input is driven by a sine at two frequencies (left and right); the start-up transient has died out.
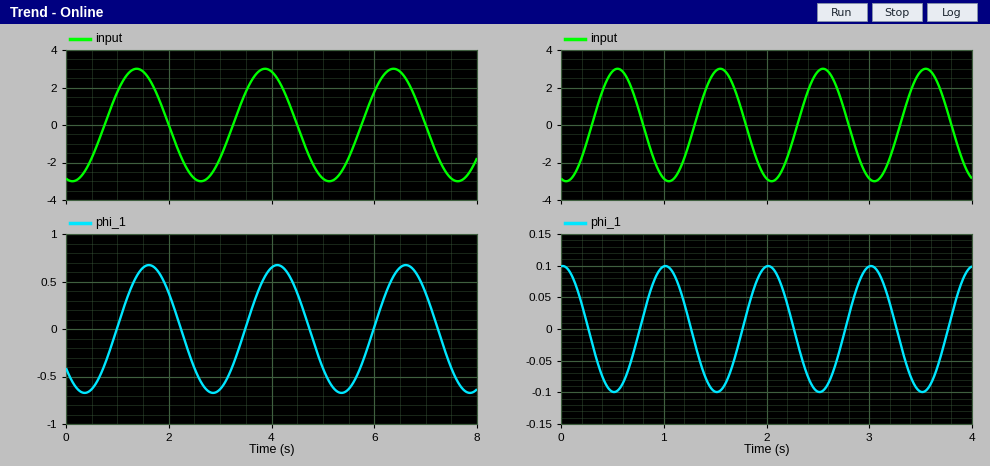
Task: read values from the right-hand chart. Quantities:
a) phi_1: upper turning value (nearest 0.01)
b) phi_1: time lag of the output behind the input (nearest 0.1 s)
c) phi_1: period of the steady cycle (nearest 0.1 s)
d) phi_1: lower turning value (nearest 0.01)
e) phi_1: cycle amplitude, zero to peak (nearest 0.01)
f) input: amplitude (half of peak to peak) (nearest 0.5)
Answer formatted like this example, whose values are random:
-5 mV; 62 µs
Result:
0.10; 0.5 s; 1.0 s; -0.10; 0.10; 3.0
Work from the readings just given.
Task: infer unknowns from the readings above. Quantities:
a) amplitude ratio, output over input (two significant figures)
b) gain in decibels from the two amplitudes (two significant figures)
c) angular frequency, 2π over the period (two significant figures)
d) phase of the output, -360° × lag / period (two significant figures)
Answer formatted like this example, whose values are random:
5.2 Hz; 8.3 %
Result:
0.033; -30 dB; 6.3 rad/s; -180°
